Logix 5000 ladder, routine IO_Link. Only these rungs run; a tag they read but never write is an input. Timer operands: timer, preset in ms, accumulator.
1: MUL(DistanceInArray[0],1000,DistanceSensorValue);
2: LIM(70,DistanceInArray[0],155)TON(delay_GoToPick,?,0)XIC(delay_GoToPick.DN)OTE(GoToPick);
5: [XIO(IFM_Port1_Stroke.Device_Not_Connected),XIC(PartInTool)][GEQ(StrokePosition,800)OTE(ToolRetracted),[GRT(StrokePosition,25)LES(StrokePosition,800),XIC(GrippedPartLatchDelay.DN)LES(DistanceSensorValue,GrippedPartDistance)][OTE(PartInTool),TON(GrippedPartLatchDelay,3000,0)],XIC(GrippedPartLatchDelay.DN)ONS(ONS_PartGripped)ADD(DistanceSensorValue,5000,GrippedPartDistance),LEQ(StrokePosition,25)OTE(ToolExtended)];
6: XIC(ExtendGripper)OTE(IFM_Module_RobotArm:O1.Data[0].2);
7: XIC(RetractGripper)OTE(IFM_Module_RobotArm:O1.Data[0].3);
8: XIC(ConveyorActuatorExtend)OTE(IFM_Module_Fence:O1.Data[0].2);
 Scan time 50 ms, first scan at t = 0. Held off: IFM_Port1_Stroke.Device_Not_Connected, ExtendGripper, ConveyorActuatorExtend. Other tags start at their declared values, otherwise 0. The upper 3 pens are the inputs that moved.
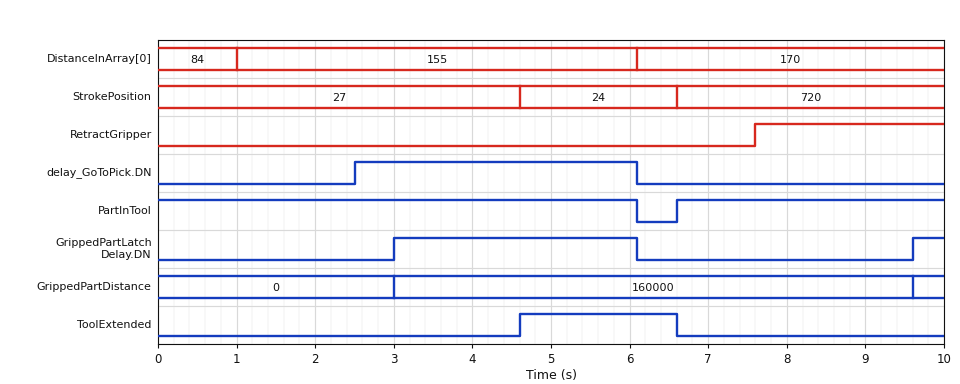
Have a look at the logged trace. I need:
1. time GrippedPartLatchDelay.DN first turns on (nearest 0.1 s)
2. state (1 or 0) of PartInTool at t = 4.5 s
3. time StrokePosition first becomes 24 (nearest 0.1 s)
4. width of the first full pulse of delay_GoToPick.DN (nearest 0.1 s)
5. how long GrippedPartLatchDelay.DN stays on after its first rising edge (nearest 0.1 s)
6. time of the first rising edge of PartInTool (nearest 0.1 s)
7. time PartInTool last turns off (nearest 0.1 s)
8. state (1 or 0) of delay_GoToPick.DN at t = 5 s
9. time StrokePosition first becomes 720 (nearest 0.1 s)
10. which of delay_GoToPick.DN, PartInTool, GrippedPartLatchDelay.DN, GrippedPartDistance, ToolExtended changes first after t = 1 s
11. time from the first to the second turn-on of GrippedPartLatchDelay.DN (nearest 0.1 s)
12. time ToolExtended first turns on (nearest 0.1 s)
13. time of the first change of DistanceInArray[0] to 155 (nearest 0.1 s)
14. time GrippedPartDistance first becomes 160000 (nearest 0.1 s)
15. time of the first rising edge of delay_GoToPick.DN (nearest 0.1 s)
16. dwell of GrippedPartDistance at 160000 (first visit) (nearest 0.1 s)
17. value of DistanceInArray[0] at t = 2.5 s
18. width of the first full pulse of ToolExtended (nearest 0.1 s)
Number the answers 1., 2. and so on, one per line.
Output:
1. 3.0 s
2. 1
3. 4.6 s
4. 3.6 s
5. 3.1 s
6. 6.6 s
7. 6.1 s
8. 1
9. 6.6 s
10. delay_GoToPick.DN
11. 6.6 s
12. 4.6 s
13. 1.0 s
14. 3.0 s
15. 2.5 s
16. 6.6 s
17. 155
18. 2.0 s
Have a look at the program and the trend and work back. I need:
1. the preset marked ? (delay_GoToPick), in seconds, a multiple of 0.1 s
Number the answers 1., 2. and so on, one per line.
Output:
1. 2.5 s
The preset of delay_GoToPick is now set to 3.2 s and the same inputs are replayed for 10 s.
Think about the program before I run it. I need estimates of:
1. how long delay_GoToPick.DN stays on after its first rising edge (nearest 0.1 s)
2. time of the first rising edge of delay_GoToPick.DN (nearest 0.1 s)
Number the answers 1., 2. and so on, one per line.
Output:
1. 2.9 s
2. 3.2 s
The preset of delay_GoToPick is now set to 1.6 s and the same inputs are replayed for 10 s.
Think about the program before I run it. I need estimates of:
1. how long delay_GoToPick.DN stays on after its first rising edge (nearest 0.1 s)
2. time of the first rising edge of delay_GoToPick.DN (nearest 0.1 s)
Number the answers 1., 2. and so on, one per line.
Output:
1. 4.5 s
2. 1.6 s
